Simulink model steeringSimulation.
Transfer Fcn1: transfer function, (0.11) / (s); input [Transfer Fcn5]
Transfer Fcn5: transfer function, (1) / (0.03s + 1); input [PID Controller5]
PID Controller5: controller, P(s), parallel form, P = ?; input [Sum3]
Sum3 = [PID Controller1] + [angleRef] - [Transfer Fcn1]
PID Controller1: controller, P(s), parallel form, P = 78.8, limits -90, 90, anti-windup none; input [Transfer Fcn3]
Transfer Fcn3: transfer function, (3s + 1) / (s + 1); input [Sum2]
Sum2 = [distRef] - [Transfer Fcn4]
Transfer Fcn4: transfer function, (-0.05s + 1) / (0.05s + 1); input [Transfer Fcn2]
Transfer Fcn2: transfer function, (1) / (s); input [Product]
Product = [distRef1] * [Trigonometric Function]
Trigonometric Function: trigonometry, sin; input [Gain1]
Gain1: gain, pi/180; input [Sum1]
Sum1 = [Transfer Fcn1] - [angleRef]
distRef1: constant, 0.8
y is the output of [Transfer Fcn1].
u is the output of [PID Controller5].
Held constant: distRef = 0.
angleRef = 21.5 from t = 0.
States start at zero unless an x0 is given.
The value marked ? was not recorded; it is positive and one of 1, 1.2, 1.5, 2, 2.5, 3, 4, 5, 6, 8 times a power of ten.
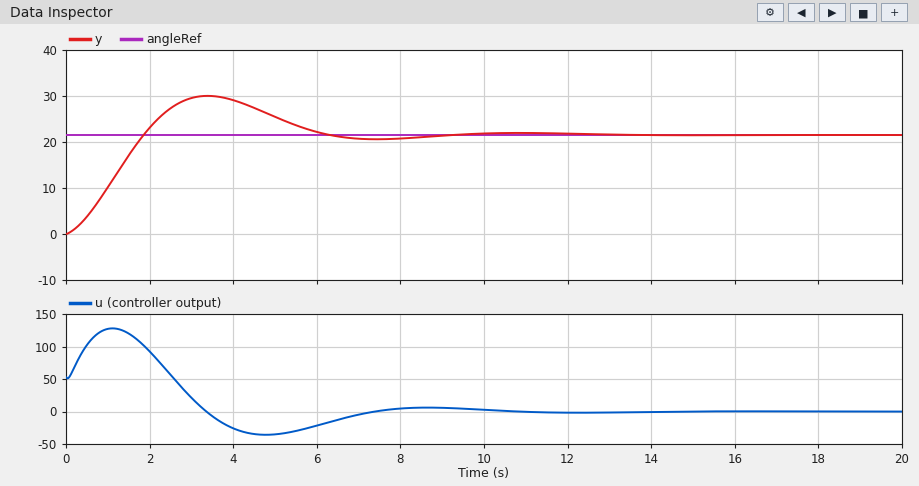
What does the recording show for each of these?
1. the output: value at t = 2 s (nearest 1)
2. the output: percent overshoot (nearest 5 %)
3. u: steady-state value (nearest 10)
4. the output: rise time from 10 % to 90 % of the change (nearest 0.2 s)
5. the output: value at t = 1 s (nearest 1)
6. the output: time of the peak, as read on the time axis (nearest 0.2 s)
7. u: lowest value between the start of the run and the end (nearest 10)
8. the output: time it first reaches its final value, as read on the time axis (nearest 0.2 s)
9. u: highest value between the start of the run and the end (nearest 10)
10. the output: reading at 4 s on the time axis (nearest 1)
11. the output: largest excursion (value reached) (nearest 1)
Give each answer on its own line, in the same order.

23
40 %
0
1.4 s
10
3.4 s
-40
1.8 s
130
29
30
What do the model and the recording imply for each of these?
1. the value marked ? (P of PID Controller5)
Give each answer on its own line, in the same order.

2.5
